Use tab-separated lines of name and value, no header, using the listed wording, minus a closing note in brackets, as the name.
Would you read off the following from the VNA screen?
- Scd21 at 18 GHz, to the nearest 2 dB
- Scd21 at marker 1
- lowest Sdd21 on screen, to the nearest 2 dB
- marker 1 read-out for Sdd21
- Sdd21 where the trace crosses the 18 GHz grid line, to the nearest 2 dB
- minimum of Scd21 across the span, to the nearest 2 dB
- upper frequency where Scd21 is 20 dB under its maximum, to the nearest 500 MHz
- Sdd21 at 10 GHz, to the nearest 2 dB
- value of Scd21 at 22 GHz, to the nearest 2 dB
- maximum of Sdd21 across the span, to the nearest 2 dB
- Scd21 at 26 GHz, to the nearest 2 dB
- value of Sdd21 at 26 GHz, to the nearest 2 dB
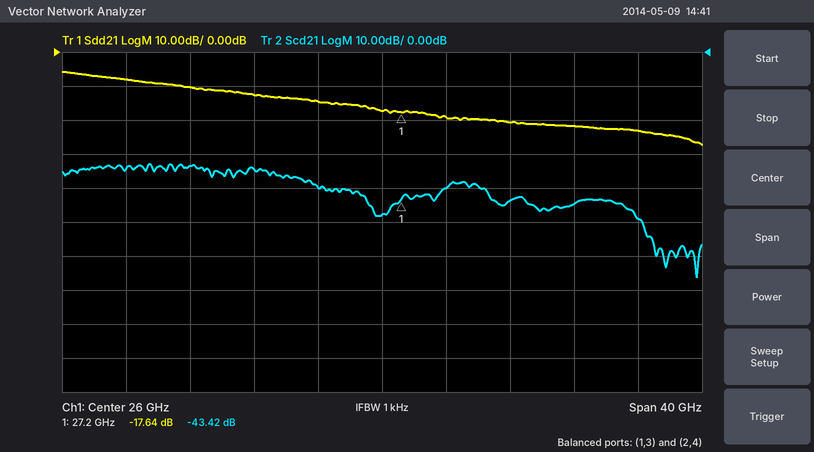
Scd21 at 18 GHz, to the nearest 2 dB	-34 dB
Scd21 at marker 1	-43.42 dB
lowest Sdd21 on screen, to the nearest 2 dB	-28 dB
marker 1 read-out for Sdd21	-17.64 dB
Sdd21 where the trace crosses the 18 GHz grid line, to the nearest 2 dB	-12 dB
minimum of Scd21 across the span, to the nearest 2 dB	-66 dB
upper frequency where Scd21 is 20 dB under its maximum, to the nearest 500 MHz	42.5 GHz
Sdd21 at 10 GHz, to the nearest 2 dB	-8 dB
value of Scd21 at 22 GHz, to the nearest 2 dB	-40 dB
maximum of Sdd21 across the span, to the nearest 2 dB	-6 dB
Scd21 at 26 GHz, to the nearest 2 dB	-48 dB
value of Sdd21 at 26 GHz, to the nearest 2 dB	-18 dB
